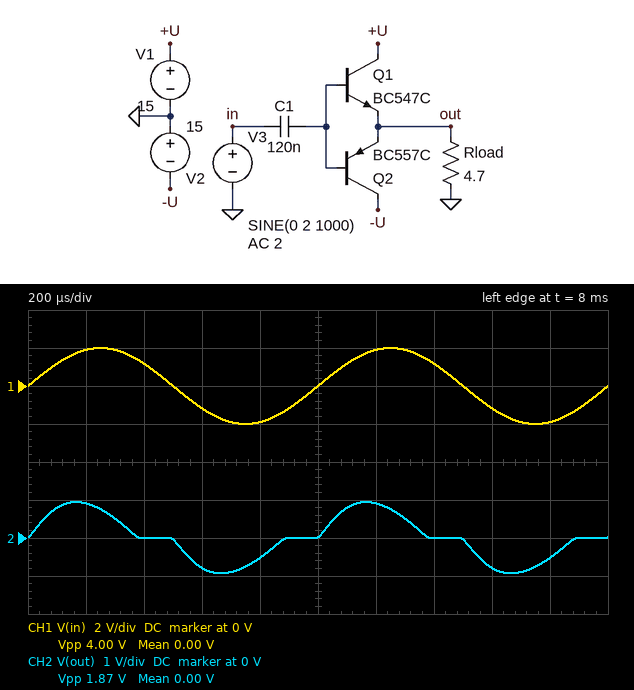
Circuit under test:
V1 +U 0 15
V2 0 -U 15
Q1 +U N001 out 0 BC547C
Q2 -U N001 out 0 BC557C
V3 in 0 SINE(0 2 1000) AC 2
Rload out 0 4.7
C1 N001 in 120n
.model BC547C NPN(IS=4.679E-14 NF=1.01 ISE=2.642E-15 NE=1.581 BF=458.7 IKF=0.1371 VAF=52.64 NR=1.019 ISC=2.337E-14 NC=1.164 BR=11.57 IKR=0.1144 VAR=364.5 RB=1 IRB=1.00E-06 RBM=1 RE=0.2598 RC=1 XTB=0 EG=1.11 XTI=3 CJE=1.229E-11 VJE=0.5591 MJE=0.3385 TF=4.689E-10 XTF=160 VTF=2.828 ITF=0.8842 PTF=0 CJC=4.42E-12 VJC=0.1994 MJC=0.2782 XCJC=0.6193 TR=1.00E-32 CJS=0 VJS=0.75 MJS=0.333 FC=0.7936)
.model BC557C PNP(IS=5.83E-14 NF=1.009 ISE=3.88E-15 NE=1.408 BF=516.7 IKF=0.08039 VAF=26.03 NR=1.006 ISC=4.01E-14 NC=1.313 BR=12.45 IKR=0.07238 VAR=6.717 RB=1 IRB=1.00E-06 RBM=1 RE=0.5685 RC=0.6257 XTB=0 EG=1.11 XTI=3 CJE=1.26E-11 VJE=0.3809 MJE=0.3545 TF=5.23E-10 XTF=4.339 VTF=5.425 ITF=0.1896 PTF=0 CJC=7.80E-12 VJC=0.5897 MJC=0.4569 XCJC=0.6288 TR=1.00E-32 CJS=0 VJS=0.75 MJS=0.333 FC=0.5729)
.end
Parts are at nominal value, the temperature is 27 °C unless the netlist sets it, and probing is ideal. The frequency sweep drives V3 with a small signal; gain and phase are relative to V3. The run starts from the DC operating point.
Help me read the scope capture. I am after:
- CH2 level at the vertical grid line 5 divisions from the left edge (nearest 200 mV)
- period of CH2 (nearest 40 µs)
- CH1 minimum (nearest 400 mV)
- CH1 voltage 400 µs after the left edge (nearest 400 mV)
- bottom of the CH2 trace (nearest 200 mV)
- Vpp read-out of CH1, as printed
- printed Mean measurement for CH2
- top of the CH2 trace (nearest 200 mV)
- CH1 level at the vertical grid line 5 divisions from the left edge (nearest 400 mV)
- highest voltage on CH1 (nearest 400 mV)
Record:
0 V
1.00 ms
-2.0 V
1.2 V
-1.0 V
4.00 V
0.00 V
1.0 V
0 V
2.0 V
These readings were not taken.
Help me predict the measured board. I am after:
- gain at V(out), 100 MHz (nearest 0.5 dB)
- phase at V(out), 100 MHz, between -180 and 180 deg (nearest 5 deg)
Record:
-22.5 dB
85 deg
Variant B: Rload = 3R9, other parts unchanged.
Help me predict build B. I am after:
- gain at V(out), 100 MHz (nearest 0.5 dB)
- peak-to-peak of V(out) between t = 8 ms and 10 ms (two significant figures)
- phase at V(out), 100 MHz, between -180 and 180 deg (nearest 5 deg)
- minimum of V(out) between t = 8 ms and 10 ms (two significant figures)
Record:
-24.5 dB
1.7 V
85 deg
-840 mV
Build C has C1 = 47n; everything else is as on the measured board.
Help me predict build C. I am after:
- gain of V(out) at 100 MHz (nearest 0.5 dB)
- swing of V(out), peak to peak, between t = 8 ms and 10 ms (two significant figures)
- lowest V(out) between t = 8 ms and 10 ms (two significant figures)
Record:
-22.5 dB
1.3 V
-670 mV
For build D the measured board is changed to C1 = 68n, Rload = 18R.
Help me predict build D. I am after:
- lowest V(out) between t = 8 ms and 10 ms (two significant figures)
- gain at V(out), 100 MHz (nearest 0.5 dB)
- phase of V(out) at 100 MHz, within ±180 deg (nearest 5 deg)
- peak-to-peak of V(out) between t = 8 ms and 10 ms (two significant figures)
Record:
-1.2 V
-11.5 dB
75 deg
2.4 V
